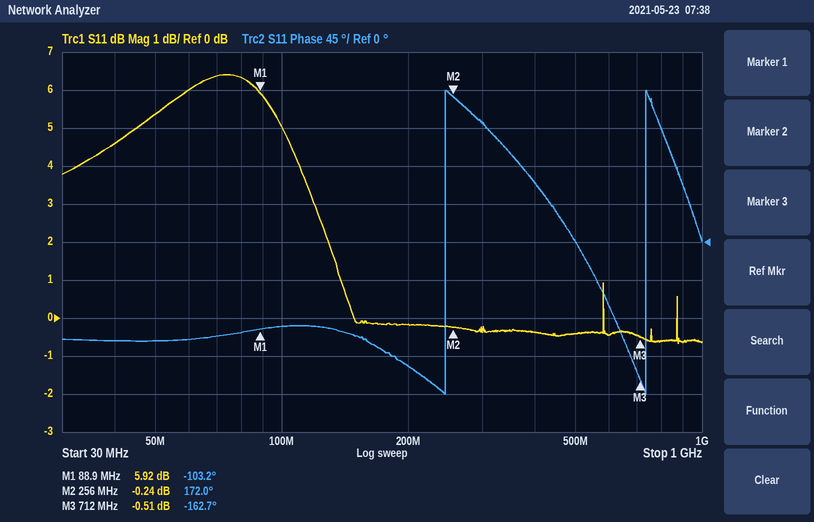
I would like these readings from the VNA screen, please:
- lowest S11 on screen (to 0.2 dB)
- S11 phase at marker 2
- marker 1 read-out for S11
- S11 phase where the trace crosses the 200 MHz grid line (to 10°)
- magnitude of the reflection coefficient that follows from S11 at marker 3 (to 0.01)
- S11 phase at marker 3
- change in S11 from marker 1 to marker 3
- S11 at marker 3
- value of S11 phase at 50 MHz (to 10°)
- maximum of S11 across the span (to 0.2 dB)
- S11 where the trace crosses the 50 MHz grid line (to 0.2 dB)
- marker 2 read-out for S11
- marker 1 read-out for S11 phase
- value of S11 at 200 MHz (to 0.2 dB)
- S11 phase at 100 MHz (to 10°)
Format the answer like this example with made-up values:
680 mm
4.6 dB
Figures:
-0.6 dB
172.0°
5.92 dB
-150°
0.94
-162.7°
-6.43 dB
-0.51 dB
-120°
6.4 dB
5.4 dB
-0.24 dB
-103.2°
-0.2 dB
-100°
